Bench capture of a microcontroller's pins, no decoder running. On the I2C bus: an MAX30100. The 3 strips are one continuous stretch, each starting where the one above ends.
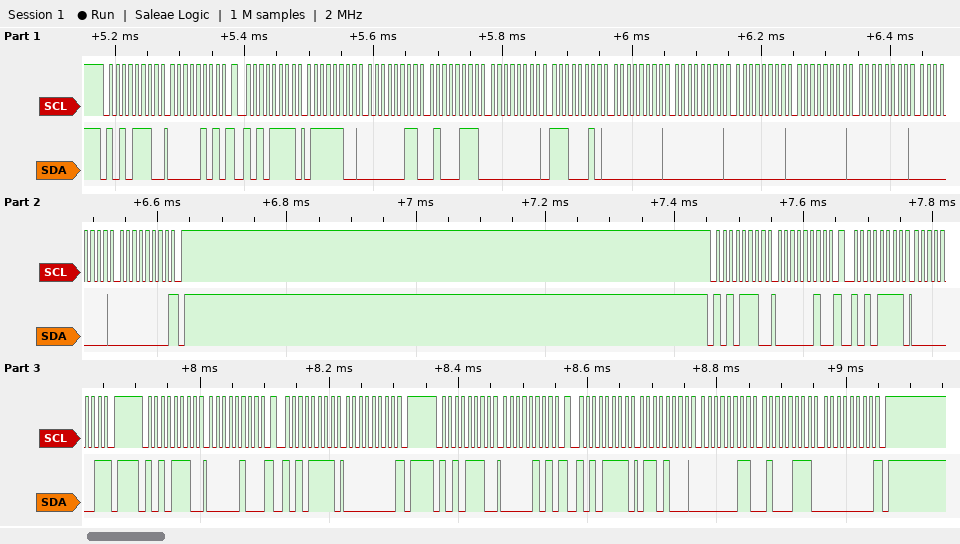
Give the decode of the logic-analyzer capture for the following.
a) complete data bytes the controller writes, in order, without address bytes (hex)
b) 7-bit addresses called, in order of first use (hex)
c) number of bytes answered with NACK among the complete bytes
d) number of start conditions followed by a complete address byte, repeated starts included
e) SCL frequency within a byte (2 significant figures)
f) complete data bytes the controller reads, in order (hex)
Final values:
05 02 04 05
0x57
4
8
100 kHz
7C 03 47 00 E2 00 00 00 00 00 00 00 01 00 68 03 47 00
